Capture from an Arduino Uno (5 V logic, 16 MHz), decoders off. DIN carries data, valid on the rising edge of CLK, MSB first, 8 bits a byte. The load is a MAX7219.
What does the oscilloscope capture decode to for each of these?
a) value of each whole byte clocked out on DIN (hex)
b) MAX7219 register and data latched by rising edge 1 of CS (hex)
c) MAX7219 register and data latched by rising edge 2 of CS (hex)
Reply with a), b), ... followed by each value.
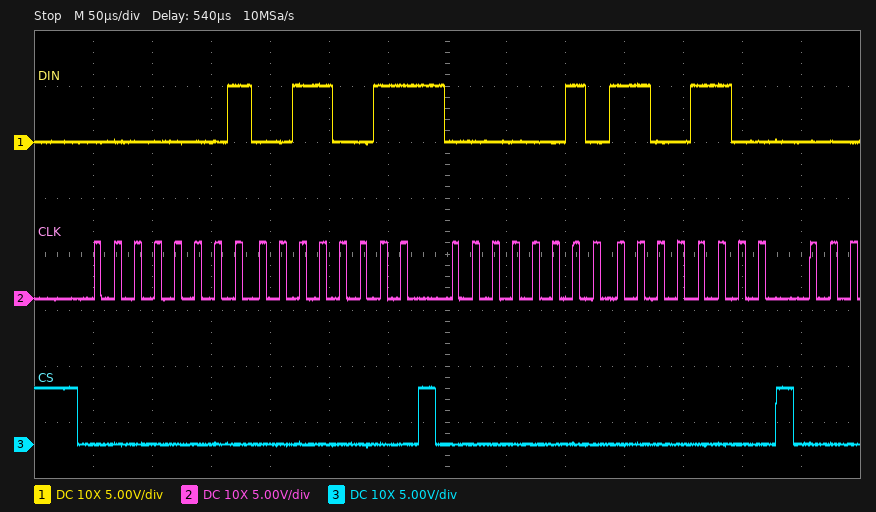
a) 01 33 02 CC
b) register 0x1, data 0x33
c) register 0x2, data 0xCC
